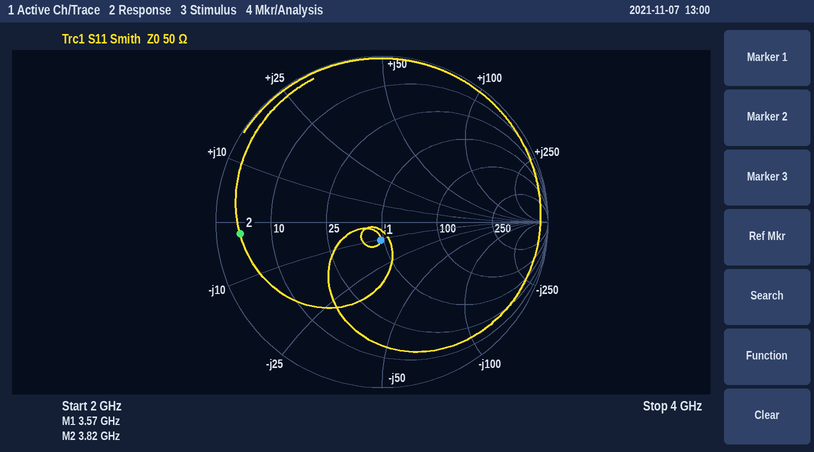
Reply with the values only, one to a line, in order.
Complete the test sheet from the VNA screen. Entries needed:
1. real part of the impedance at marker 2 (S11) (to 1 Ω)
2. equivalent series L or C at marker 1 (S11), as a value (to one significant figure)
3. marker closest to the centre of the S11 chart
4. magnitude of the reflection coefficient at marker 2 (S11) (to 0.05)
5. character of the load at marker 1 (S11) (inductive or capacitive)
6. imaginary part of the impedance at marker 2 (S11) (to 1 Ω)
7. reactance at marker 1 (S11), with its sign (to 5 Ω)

4 Ω
4 pF
marker 1
0.85
capacitive
-2 Ω
-10 Ω
